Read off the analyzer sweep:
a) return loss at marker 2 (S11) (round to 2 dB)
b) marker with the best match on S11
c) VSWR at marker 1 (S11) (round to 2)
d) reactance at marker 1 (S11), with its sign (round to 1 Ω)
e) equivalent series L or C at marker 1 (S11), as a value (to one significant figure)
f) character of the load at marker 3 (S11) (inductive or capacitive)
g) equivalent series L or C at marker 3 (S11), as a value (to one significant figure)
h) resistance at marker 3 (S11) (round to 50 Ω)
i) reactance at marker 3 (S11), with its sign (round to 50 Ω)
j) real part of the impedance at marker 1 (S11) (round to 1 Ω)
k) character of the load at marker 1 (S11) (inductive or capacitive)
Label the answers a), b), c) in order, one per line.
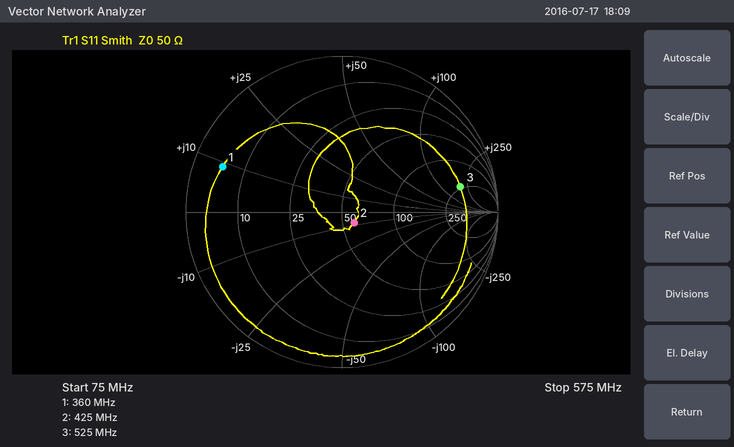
a) 20 dB
b) marker 2
c) 10
d) +9 Ω
e) 4 nH
f) inductive
g) 60 nH
h) 250 Ω
i) +200 Ω
j) 5 Ω
k) inductive
